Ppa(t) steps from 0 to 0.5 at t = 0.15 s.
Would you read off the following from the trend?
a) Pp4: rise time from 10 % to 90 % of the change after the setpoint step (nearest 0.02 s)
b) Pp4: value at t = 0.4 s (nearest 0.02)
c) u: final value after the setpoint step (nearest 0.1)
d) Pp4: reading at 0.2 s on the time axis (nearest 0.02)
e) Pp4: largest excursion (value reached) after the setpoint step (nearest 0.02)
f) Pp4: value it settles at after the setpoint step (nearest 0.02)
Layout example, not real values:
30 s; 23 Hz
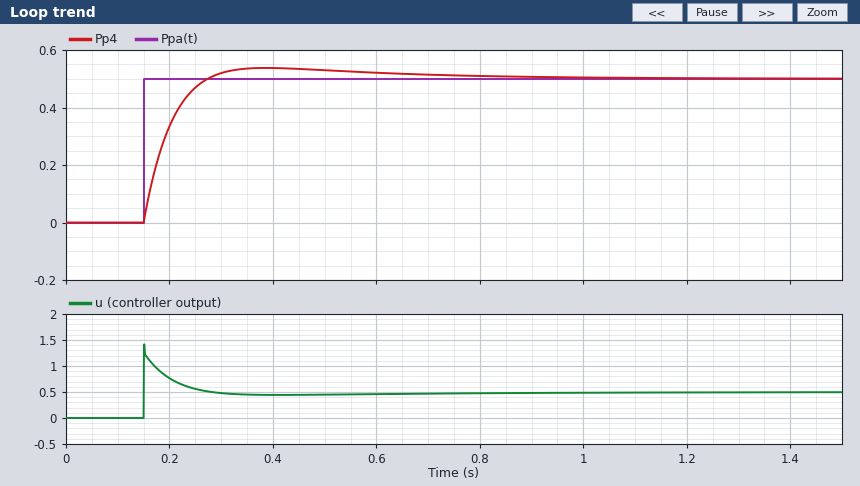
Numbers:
0.08 s; 0.54; 0.5; 0.34; 0.54; 0.50
